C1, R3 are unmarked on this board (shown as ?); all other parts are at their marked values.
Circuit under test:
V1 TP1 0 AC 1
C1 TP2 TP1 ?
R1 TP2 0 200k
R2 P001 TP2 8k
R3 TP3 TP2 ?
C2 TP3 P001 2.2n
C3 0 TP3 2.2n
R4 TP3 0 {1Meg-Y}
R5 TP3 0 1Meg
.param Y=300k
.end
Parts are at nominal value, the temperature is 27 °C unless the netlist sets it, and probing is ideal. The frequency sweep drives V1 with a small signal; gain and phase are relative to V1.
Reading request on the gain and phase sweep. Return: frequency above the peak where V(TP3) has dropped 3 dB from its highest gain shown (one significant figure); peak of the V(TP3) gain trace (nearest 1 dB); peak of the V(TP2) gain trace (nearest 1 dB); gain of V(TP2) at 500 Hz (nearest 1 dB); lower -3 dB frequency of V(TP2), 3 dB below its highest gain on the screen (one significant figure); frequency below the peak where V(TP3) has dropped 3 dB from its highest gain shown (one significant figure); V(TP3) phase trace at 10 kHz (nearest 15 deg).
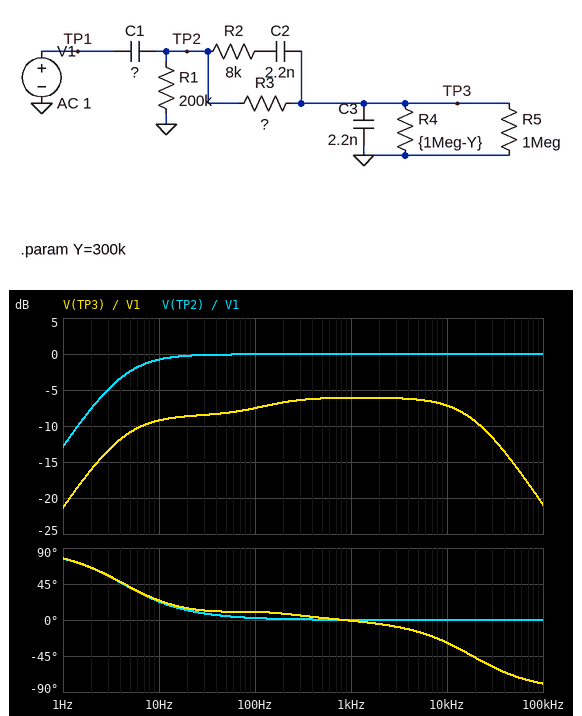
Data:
20 kHz
-6 dB
0 dB
0 dB
4 Hz
10 Hz
-30 deg
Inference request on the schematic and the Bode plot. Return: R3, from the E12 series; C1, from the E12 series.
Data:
680 kΩ
220 nF
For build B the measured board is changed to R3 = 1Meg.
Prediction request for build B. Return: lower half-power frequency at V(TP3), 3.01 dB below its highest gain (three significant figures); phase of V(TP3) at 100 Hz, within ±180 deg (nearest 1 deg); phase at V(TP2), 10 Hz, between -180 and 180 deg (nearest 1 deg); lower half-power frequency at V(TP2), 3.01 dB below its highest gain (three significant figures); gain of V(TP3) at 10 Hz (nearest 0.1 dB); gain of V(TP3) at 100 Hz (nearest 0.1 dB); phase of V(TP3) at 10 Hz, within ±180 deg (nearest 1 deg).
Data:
68.9 Hz
17 deg
22 deg
4.15 Hz
-11.4 dB
-8.3 dB
26 deg
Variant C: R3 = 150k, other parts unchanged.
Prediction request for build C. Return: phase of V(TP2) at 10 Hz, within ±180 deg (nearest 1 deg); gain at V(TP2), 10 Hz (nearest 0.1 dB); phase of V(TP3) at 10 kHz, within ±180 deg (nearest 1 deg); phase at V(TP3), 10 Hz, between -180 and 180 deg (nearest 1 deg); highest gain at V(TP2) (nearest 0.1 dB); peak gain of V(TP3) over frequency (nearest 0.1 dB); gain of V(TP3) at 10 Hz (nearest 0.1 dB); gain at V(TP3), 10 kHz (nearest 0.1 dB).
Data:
26 deg
-1.0 dB
-29 deg
25 deg
0 dB
-2.8 dB
-3.7 dB
-6.9 dB
